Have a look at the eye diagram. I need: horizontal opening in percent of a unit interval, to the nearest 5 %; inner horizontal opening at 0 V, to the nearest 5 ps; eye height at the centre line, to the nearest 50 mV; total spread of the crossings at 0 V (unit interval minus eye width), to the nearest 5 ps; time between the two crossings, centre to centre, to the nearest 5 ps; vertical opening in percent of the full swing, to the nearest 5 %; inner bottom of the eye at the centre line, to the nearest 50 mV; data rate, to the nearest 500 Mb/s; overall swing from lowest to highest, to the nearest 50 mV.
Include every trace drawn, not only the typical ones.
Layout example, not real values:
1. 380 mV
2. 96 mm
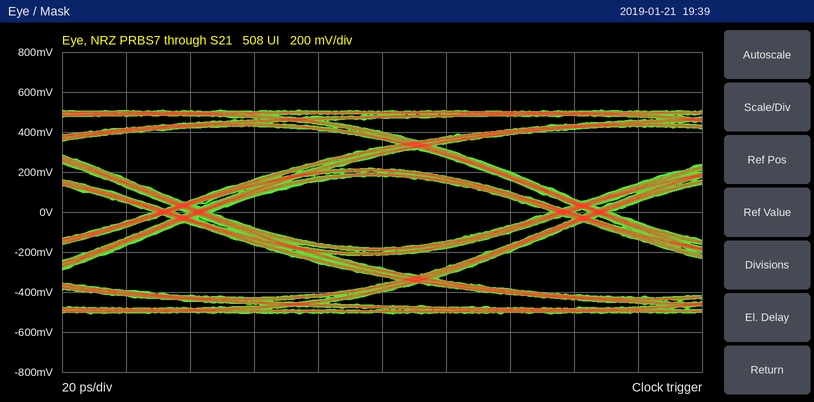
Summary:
1. 85 %
2. 105 ps
3. 350 mV
4. 20 ps
5. 125 ps
6. 35 %
7. -200 mV
8. 8.0 Gb/s
9. 1.00 V
